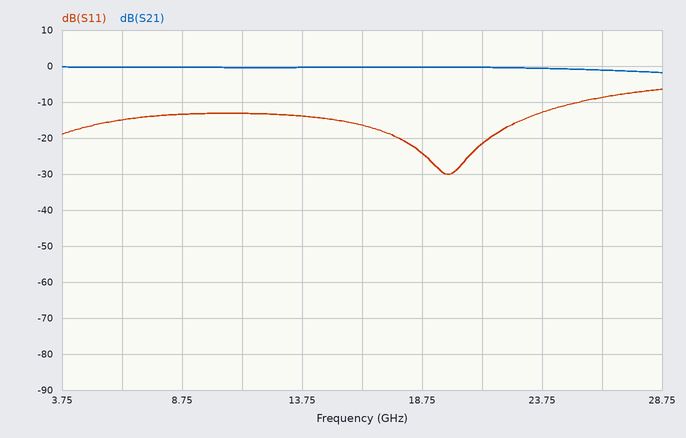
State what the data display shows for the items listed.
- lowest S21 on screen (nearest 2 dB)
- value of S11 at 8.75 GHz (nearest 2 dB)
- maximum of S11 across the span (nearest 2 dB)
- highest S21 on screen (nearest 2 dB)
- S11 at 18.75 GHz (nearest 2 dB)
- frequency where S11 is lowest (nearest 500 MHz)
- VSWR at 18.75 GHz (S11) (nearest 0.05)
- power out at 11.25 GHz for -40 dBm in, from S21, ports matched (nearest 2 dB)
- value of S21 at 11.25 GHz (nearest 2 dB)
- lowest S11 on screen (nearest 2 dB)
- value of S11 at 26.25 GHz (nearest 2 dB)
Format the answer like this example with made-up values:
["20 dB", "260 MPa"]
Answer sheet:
["-2 dB", "-14 dB", "-6 dB", "0 dB", "-24 dB", "20.0 GHz", "1.15", "-40 dBm", "0 dB", "-30 dB", "-8 dB"]
